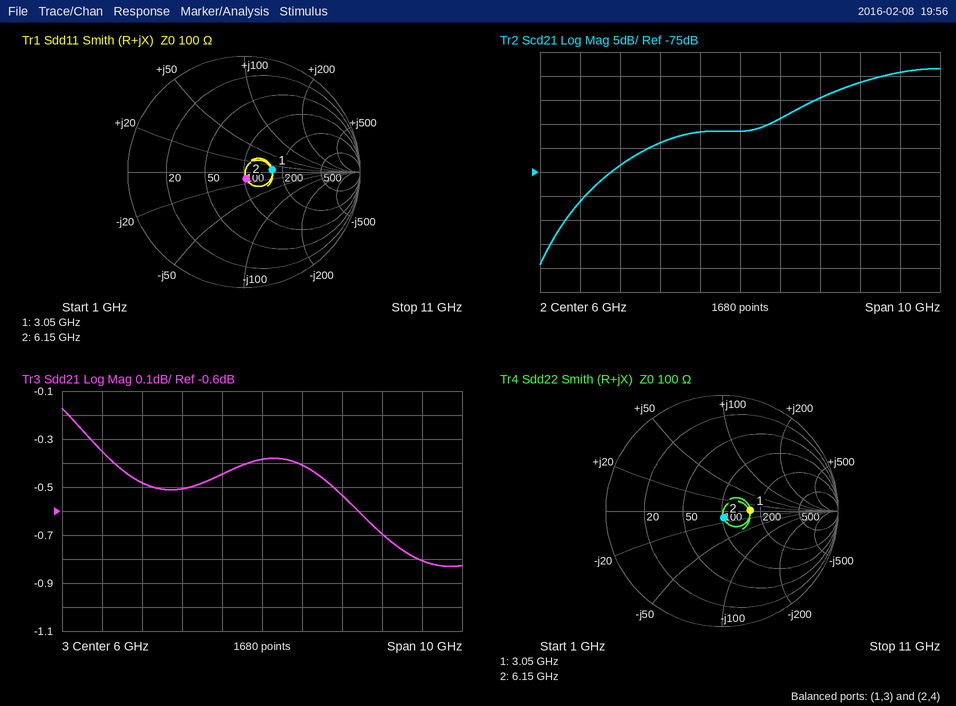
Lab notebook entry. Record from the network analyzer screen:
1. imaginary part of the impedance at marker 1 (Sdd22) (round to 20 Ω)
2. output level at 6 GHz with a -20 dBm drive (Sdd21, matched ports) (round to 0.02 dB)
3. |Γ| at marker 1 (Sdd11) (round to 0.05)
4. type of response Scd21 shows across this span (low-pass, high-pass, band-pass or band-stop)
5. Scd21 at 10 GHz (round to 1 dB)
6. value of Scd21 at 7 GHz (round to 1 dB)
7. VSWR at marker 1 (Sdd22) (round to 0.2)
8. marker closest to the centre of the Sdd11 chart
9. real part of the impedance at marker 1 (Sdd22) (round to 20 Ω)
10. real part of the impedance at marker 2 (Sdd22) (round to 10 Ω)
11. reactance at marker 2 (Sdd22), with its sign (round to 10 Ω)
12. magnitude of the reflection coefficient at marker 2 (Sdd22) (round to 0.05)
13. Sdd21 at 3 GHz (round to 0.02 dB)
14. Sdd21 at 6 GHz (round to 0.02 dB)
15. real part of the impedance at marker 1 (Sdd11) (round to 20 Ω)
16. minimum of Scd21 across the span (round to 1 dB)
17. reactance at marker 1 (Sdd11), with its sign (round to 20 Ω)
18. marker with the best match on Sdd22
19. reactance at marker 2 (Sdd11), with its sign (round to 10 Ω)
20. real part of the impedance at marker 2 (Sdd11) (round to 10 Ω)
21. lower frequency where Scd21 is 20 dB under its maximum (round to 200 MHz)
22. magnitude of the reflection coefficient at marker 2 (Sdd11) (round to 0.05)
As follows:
0 Ω
-20.38 dBm
0.25
high-pass
-54 dB
-64 dB
1.6
marker 2
160 Ω
100 Ω
-10 Ω
0.05
-0.48 dB
-0.38 dB
160 Ω
-94 dB
0 Ω
marker 2
-10 Ω
100 Ω
3.0 GHz
0.05
